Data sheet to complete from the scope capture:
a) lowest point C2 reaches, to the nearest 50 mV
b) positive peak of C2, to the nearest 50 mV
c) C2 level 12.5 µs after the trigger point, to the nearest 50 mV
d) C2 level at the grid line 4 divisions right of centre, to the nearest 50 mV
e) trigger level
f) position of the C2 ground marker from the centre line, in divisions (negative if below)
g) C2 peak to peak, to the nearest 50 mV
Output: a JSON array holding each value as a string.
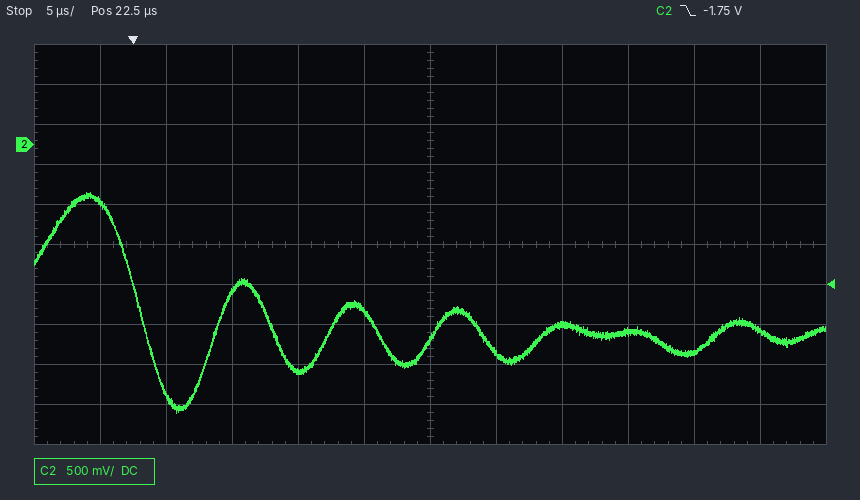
["-3.35 V", "-600 mV", "-2.85 V", "-2.60 V", "-1.75 V", "+2.5 div", "2.75 V"]
